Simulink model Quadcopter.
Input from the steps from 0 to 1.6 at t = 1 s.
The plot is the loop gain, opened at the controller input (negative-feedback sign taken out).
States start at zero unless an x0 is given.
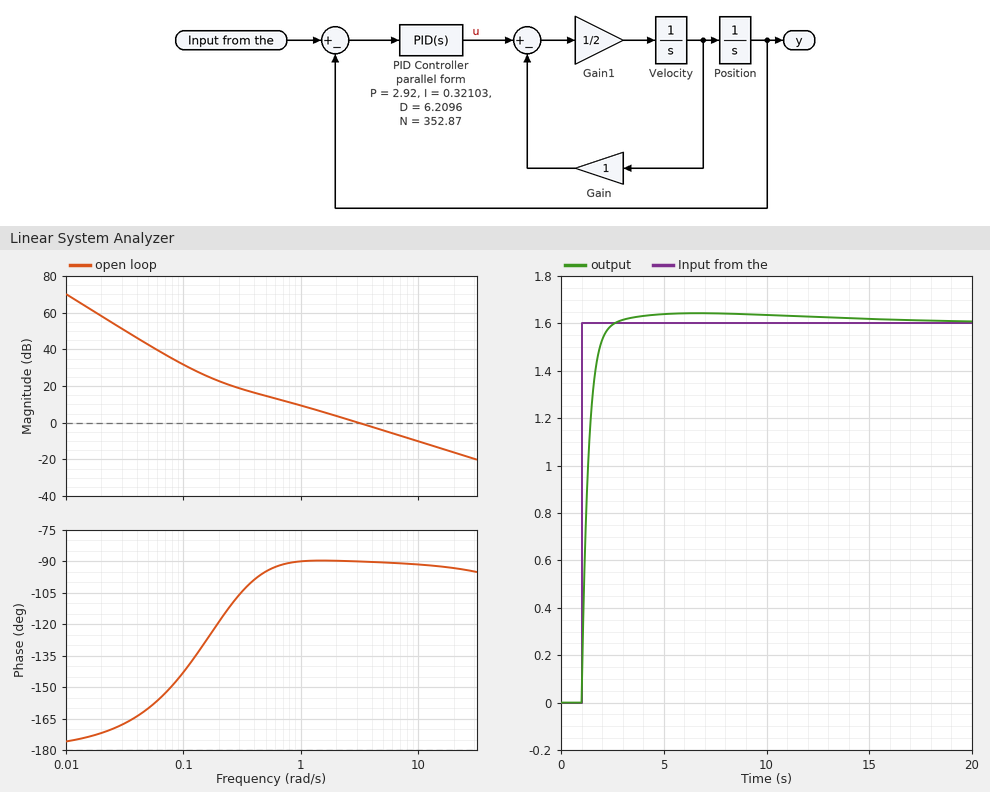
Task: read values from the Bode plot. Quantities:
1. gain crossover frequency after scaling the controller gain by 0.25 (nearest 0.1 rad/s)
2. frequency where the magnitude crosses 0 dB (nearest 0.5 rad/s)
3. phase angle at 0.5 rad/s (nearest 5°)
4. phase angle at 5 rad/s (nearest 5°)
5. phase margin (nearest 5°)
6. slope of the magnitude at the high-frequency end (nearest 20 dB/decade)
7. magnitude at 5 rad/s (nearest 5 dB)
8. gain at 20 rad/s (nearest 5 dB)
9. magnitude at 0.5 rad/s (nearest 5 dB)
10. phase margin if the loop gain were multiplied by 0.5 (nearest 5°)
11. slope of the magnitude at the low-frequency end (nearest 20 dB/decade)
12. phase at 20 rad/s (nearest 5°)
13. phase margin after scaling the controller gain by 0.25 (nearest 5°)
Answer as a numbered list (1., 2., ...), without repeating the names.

1. 0.7 rad/s
2. 3.0 rad/s
3. -95°
4. -90°
5. 90°
6. -20 dB/decade
7. -5 dB
8. -15 dB
9. 15 dB
10. 90°
11. -40 dB/decade
12. -95°
13. 90°
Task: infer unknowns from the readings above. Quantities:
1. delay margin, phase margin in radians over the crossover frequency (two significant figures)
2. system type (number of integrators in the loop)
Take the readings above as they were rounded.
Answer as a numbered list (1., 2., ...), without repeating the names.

1. 0.52 s
2. 2
